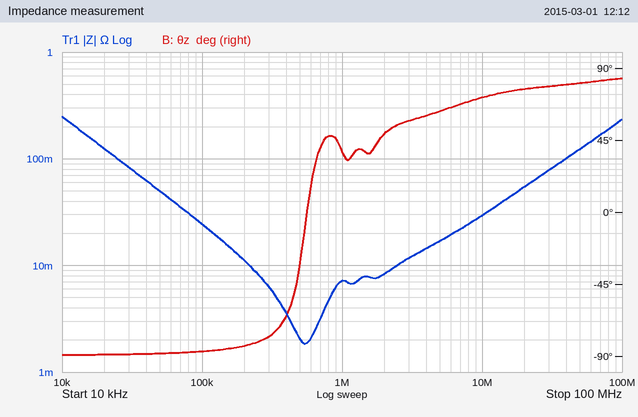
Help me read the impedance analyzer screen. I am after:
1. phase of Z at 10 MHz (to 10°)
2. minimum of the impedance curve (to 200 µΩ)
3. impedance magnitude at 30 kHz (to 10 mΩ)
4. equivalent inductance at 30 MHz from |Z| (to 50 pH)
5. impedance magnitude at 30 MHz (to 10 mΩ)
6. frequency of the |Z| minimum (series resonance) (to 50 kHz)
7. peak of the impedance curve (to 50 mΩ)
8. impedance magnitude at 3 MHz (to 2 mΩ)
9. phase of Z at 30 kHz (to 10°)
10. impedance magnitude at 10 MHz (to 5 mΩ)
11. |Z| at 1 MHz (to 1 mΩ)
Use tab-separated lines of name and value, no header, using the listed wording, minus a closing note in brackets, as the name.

phase of Z at 10 MHz	70°
minimum of the impedance curve	1.8 mΩ
impedance magnitude at 30 kHz	80 mΩ
equivalent inductance at 30 MHz from |Z|	400 pH
impedance magnitude at 30 MHz	80 mΩ
frequency of the |Z| minimum (series resonance)	550 kHz
peak of the impedance curve	250 mΩ
impedance magnitude at 3 MHz	12 mΩ
phase of Z at 30 kHz	-90°
impedance magnitude at 10 MHz	30 mΩ
|Z| at 1 MHz	7 mΩ
